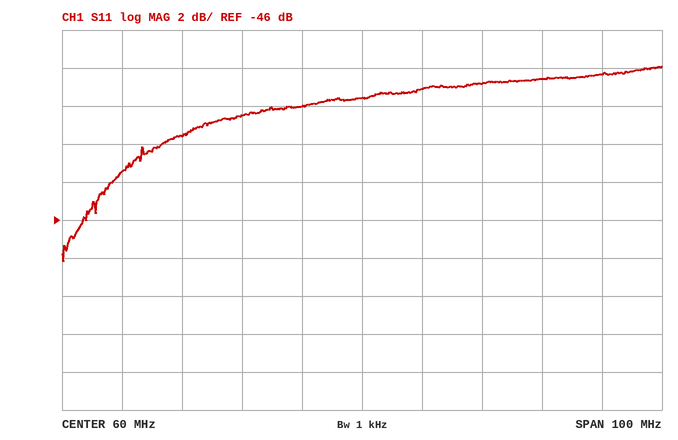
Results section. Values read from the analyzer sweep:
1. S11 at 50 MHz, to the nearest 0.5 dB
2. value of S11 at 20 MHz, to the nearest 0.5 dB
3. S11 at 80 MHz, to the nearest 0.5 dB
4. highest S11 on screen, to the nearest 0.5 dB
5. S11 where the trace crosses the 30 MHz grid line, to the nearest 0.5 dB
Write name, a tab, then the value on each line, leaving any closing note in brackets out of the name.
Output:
S11 at 50 MHz, to the nearest 0.5 dB	-40.0 dB
value of S11 at 20 MHz, to the nearest 0.5 dB	-43.5 dB
S11 at 80 MHz, to the nearest 0.5 dB	-39.0 dB
highest S11 on screen, to the nearest 0.5 dB	-38.0 dB
S11 where the trace crosses the 30 MHz grid line, to the nearest 0.5 dB	-41.5 dB
